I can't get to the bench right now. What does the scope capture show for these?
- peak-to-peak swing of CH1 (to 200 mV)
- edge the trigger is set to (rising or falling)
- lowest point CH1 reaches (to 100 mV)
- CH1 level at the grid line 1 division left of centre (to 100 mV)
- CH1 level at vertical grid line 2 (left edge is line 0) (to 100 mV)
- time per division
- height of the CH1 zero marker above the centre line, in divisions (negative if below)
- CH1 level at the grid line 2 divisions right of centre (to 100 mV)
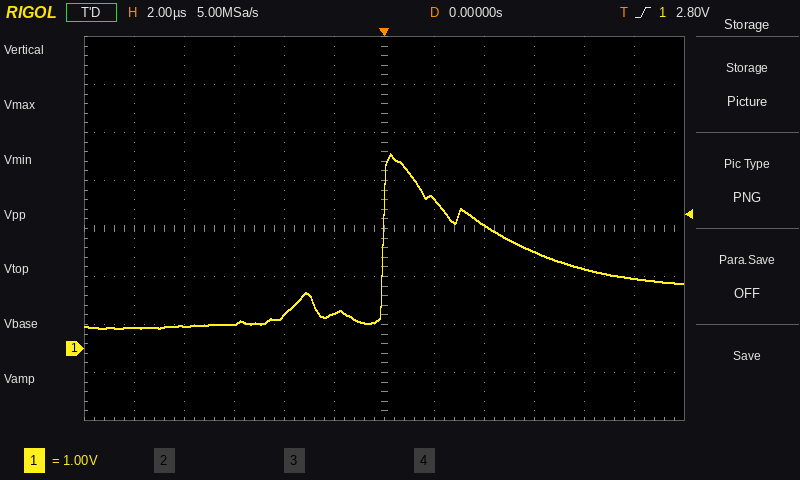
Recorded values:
3.6 V
rising
400 mV
700 mV
500 mV
2 µs
-2.5 div
2.6 V
